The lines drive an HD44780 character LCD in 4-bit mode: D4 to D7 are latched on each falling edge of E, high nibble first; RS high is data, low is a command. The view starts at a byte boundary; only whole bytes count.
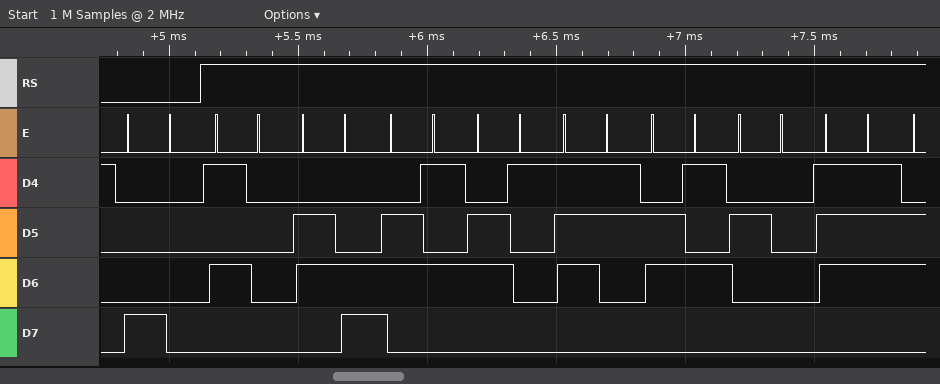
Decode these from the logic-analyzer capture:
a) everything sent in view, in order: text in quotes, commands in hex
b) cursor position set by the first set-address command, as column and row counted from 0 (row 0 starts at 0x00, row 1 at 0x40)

0x80 "Please w"
column 0, row 0
